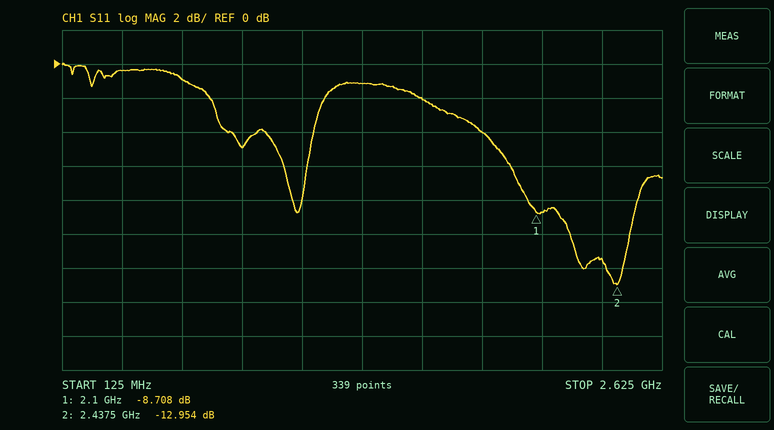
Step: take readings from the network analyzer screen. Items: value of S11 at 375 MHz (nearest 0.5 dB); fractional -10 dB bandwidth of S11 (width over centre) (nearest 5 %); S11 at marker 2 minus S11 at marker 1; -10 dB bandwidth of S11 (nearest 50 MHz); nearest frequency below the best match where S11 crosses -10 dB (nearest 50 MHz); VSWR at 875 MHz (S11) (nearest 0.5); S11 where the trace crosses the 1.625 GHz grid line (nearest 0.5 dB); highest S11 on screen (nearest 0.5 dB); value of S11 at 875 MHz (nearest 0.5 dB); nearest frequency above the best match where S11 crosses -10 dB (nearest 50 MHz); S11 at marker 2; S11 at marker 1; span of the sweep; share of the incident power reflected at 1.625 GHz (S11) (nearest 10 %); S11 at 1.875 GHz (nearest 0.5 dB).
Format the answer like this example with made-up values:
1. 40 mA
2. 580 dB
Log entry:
1. -0.5 dB
2. 10 %
3. -4.246 dB
4. 250 MHz
5. 2.25 GHz
6. 3.5
7. -2.0 dB
8. 0.0 dB
9. -5.0 dB
10. 2.50 GHz
11. -12.954 dB
12. -8.708 dB
13. 2.5 GHz
14. 60 %
15. -4.0 dB
